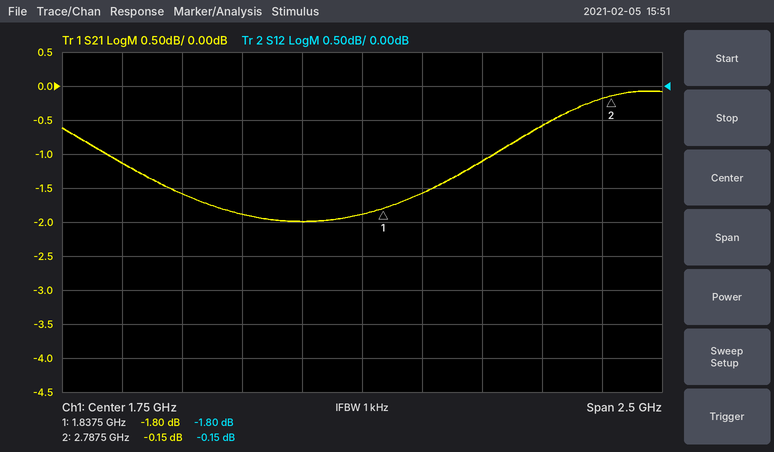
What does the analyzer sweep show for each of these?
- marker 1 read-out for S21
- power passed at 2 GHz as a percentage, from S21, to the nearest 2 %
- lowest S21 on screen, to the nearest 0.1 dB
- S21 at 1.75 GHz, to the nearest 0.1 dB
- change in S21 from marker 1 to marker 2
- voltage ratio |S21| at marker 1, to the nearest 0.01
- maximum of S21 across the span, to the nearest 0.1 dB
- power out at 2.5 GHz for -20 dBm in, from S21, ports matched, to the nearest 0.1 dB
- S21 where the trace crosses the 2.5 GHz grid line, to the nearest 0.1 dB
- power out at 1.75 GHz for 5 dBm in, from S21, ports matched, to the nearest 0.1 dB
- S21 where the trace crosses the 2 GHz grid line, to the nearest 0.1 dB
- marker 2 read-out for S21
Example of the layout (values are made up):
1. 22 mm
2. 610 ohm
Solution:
1. -1.80 dB
2. 70 %
3. -2.0 dB
4. -1.9 dB
5. 1.65 dB
6. 0.81
7. -0.1 dB
8. -20.6 dBm
9. -0.6 dB
10. 3.1 dBm
11. -1.6 dB
12. -0.15 dB
